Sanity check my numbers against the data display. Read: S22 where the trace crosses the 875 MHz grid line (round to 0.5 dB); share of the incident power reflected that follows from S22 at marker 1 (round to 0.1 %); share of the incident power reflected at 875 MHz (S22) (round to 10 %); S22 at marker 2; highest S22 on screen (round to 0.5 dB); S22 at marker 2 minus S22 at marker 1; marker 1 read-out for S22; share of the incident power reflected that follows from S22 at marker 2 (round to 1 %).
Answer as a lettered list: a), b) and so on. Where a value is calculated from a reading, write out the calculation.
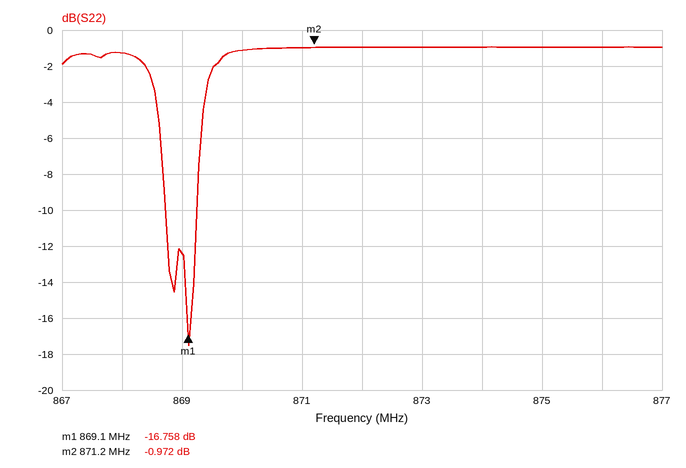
a) -1.0 dB
b) 10^(-16.758/10) ≈ 2.1 %
c) 10^(-1/10) ≈ 79.4 %, so 80 % to the nearest 10 %
d) -0.972 dB
e) -1.0 dB
f) -0.972 − (-16.758) = 15.786 dB
g) -16.758 dB
h) 10^(-0.972/10) ≈ 80 %
